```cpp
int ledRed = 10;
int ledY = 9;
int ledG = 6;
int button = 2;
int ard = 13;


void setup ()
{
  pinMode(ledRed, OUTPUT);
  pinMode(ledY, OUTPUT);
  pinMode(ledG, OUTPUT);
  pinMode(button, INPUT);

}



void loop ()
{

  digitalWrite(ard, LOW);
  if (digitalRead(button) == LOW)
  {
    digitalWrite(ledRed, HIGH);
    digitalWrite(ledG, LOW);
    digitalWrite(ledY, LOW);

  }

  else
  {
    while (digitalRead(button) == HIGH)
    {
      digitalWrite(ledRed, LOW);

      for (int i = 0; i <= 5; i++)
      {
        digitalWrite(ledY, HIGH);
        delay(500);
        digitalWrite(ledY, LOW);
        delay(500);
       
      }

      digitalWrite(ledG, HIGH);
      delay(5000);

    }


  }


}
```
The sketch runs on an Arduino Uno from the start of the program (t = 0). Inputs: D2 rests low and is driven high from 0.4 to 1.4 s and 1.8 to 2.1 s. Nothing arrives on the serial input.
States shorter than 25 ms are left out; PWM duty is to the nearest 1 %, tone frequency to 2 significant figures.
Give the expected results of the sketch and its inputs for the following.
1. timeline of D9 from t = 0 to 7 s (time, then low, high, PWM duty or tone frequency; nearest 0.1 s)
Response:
0 s low; 0.4 s high; 0.9 s low; 1.4 s high; 1.9 s low; 2.4 s high; 2.9 s low; 3.4 s high; 3.9 s low; 4.4 s high; 4.9 s low; 5.4 s high; 5.9 s low
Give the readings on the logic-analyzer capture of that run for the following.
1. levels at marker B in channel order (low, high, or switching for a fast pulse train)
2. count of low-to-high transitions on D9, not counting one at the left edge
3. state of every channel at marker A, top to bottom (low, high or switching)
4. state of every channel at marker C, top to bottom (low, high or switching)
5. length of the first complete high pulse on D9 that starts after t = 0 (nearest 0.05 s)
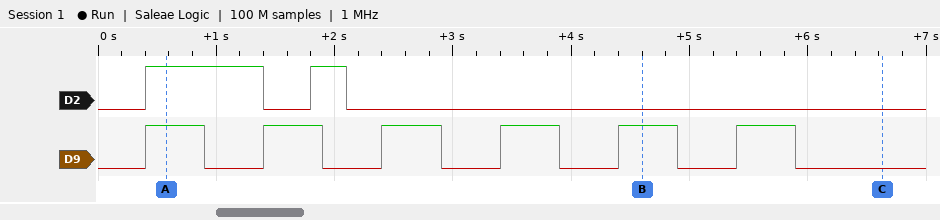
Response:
D2 low, D9 high
6
D2 high, D9 high
D2 low, D9 low
0.50 s
